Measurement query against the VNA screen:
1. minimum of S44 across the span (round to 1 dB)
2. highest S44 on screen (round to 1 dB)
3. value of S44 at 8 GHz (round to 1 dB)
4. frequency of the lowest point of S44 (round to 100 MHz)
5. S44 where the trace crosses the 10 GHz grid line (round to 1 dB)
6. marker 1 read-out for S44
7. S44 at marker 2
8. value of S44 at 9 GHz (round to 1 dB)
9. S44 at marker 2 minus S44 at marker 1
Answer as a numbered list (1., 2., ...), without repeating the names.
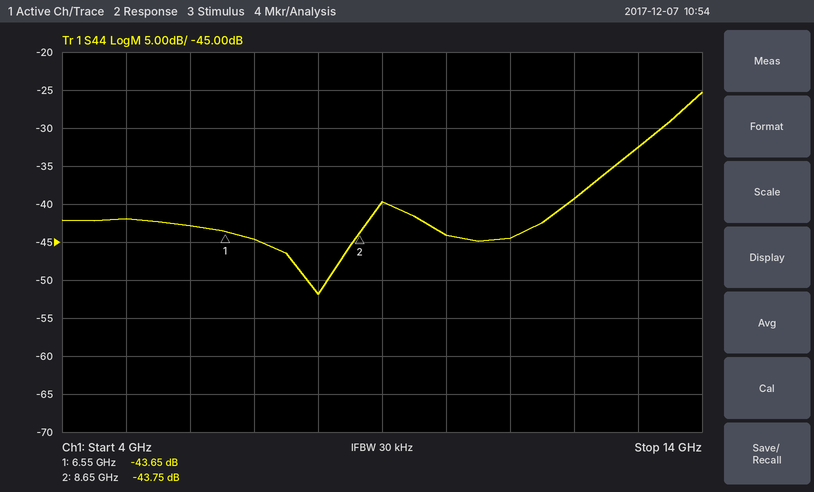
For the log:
1. -52 dB
2. -25 dB
3. -52 dB
4. 8.0 GHz
5. -44 dB
6. -43.65 dB
7. -43.75 dB
8. -40 dB
9. -0.10 dB
